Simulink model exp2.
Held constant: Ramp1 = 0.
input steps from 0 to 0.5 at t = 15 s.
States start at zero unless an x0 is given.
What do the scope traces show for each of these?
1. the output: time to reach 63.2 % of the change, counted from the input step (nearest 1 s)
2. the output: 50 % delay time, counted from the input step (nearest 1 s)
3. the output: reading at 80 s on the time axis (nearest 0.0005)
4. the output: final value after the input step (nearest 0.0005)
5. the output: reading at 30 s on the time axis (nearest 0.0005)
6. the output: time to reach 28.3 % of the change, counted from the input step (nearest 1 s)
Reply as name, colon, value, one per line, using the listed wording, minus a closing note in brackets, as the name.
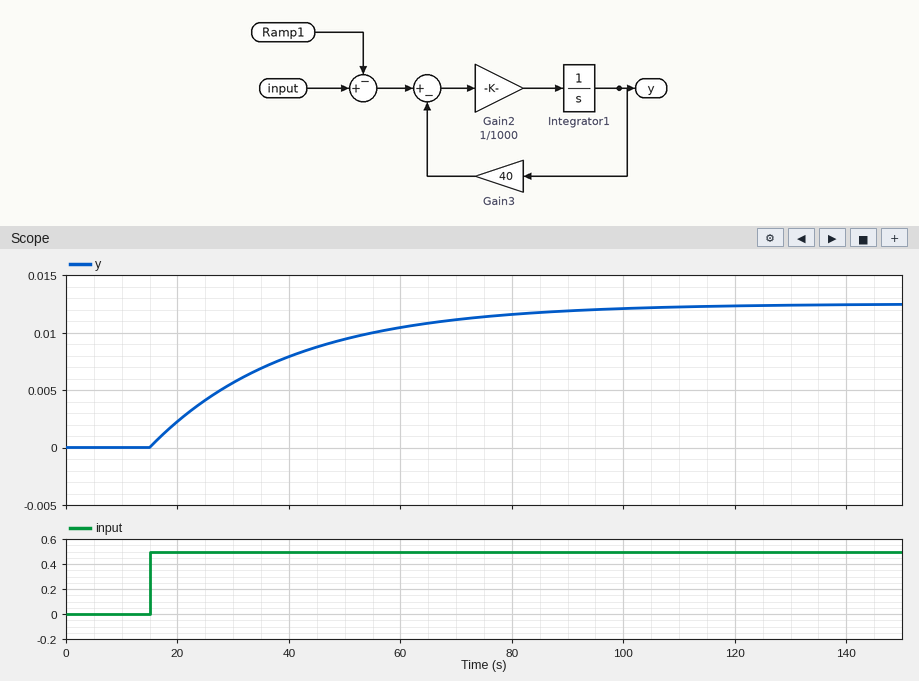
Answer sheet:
the output: time to reach 63.2 % of the change, counted from the input step: 25 s
the output: 50 % delay time, counted from the input step: 17 s
the output: reading at 80 s on the time axis: 0.0115
the output: final value after the input step: 0.0125
the output: reading at 30 s on the time axis: 0.0055
the output: time to reach 28.3 % of the change, counted from the input step: 8 s
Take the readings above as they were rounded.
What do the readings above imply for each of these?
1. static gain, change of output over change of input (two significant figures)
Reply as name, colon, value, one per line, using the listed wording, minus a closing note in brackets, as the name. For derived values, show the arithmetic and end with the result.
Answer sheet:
static gain, change of output over change of input: (0.0125 - 0) / (0.5 - 0) = 0.025
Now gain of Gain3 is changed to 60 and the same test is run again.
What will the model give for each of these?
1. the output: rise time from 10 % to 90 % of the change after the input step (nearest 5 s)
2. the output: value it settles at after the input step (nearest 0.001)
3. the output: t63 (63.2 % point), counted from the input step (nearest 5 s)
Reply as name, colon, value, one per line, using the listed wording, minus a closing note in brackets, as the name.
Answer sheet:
the output: rise time from 10 % to 90 % of the change after the input step: 35 s
the output: value it settles at after the input step: 0.008
the output: t63 (63.2 % point), counted from the input step: 15 s
